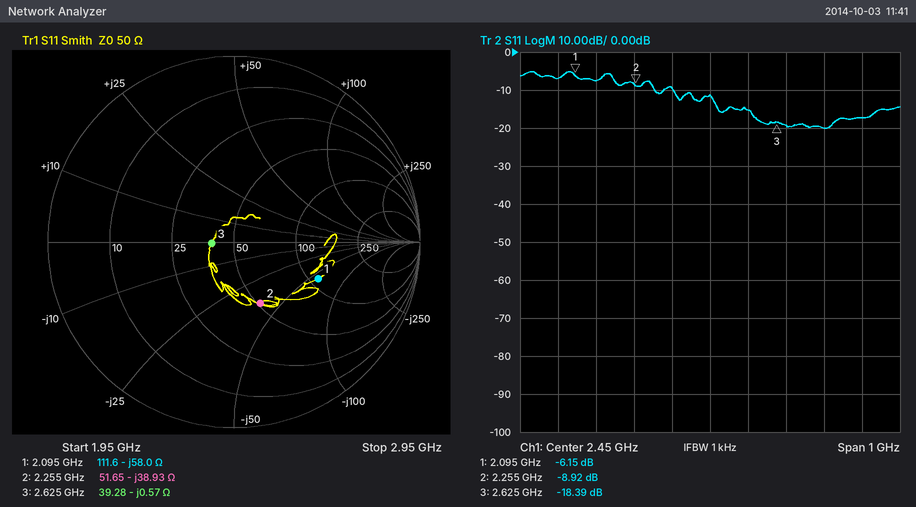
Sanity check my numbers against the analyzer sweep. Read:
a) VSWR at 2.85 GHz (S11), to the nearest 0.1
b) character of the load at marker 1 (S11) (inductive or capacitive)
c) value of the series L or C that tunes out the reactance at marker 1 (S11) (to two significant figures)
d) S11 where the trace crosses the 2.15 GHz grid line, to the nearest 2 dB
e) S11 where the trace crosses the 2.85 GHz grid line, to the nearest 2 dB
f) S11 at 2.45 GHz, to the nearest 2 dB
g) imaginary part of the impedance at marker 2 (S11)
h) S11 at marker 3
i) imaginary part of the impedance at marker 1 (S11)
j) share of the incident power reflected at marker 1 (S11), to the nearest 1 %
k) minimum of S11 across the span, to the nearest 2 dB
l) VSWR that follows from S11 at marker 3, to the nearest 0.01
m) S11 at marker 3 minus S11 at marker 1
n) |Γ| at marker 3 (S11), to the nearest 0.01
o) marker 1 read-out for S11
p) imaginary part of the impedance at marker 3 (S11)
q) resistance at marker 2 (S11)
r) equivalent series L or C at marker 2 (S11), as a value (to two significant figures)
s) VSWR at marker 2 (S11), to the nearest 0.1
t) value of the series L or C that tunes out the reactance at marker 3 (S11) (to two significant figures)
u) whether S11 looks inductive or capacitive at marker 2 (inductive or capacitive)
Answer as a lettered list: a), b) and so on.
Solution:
a) 1.3
b) capacitive
c) 4.4 nH
d) -8 dB
e) -18 dB
f) -12 dB
g) -38.93 Ω
h) -18.39 dB
i) -58.0 Ω
j) 24 %
k) -20 dB
l) 1.27
m) -12.24 dB
n) 0.12
o) -6.15 dB
p) -0.57 Ω
q) 51.65 Ω
r) 1.8 pF
s) 2.1
t) 35 pH
u) capacitive
